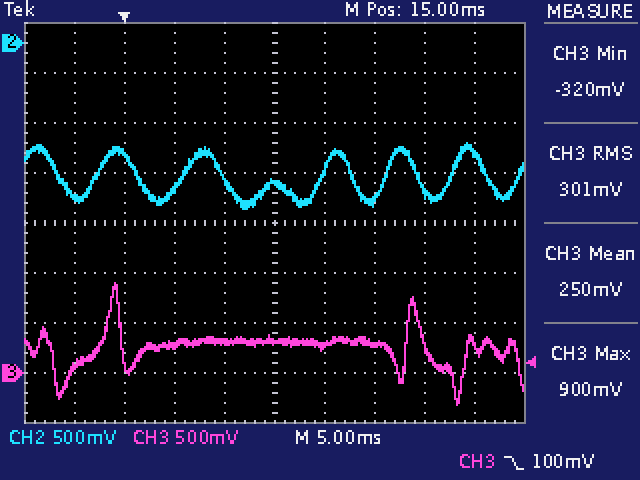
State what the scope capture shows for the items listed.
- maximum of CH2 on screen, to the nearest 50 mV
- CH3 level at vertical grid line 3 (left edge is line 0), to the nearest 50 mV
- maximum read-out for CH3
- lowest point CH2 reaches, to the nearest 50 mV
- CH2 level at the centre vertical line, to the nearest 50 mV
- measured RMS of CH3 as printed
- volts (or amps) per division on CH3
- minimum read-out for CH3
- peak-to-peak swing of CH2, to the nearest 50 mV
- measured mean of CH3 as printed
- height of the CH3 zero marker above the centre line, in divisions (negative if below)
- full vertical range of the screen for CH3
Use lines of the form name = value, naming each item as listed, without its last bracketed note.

maximum of CH2 on screen, to the nearest 50 mV = -1.00 V
CH3 level at vertical grid line 3 (left edge is line 0), to the nearest 50 mV = 300 mV
maximum read-out for CH3 = 900 mV
lowest point CH2 reaches, to the nearest 50 mV = -1.65 V
CH2 level at the centre vertical line, to the nearest 50 mV = -1.40 V
measured RMS of CH3 as printed = 301 mV
volts (or amps) per division on CH3 = 500 mV
minimum read-out for CH3 = -320 mV
peak-to-peak swing of CH2, to the nearest 50 mV = 650 mV
measured mean of CH3 as printed = 250 mV
height of the CH3 zero marker above the centre line, in divisions = -3.0 div
full vertical range of the screen for CH3 = 4 V
